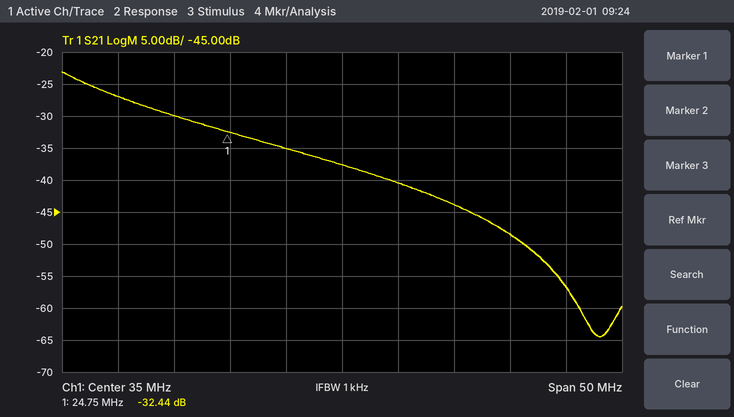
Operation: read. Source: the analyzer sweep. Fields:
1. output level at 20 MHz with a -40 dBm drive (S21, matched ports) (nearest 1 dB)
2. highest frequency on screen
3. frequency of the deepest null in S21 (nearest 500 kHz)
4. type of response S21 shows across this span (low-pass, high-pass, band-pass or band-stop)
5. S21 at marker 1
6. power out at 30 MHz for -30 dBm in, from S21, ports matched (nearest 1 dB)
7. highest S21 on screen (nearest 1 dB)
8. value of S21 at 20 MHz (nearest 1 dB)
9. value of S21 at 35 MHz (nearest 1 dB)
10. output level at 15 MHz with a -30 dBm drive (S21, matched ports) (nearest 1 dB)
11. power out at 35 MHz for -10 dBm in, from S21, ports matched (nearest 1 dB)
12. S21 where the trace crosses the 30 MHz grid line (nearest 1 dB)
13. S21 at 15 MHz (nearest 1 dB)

-70 dBm
60 MHz
58.0 MHz
low-pass
-32.44 dB
-65 dBm
-23 dB
-30 dB
-38 dB
-57 dBm
-48 dBm
-35 dB
-27 dB
